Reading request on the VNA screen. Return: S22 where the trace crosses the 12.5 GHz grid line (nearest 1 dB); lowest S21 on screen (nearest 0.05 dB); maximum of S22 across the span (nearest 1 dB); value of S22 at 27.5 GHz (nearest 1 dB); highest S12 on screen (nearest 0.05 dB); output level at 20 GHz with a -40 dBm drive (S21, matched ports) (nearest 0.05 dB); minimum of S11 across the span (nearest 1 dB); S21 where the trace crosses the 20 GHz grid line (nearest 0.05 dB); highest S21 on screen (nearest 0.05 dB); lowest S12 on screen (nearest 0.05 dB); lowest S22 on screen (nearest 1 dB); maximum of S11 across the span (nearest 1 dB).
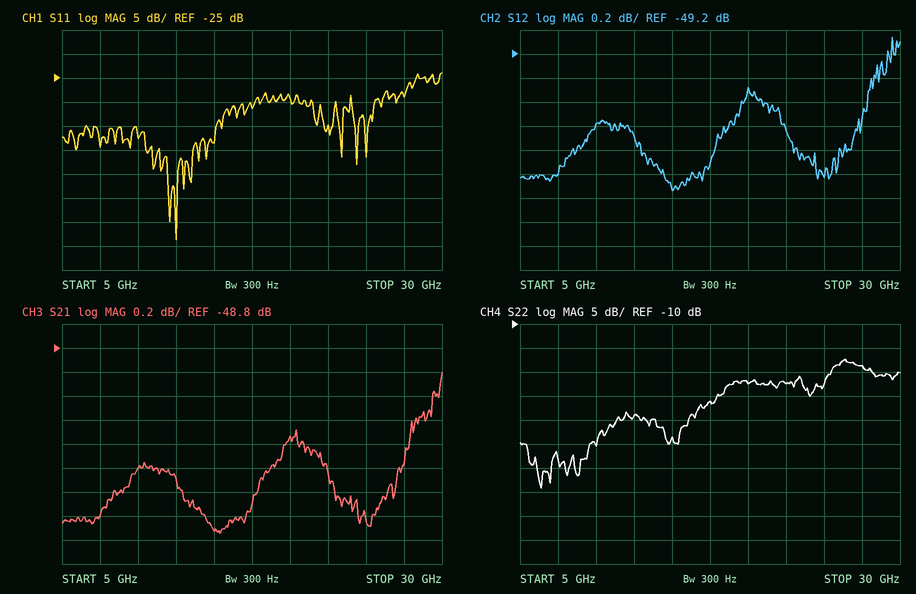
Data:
-29 dB
-50.35 dB
-17 dB
-19 dB
-49.05 dB
-89.55 dBm
-59 dB
-49.55 dB
-49.00 dB
-50.35 dB
-44 dB
-24 dB
